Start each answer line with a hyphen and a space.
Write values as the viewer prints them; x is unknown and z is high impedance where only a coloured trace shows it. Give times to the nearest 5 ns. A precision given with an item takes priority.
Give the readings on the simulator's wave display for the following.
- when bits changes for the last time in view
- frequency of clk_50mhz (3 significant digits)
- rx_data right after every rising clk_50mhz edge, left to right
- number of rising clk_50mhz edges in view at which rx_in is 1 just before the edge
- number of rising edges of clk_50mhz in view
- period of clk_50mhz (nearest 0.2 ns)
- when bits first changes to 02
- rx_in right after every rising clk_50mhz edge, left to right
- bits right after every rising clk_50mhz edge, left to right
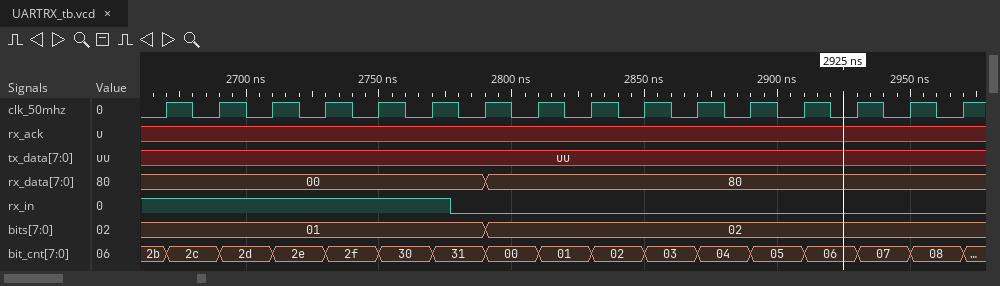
- 2790 ns
- 50.0 MHz
- 00, 00, 00, 00, 00, 00, 80, 80, 80, 80, 80, 80, 80, 80, 80, 80
- 6
- 16
- 20 ns
- 2790 ns
- 1 1 1 1 1 1 0 0 0 0 0 0 0 0 0 0
- 01, 01, 01, 01, 01, 01, 02, 02, 02, 02, 02, 02, 02, 02, 02, 02
